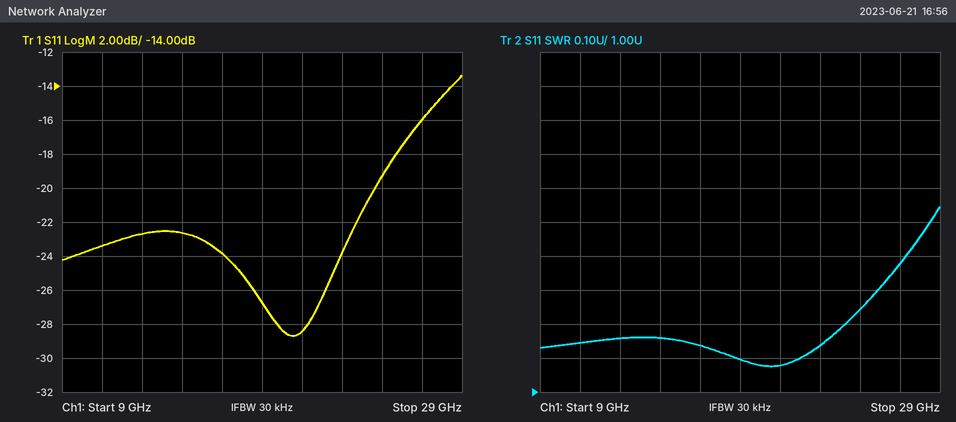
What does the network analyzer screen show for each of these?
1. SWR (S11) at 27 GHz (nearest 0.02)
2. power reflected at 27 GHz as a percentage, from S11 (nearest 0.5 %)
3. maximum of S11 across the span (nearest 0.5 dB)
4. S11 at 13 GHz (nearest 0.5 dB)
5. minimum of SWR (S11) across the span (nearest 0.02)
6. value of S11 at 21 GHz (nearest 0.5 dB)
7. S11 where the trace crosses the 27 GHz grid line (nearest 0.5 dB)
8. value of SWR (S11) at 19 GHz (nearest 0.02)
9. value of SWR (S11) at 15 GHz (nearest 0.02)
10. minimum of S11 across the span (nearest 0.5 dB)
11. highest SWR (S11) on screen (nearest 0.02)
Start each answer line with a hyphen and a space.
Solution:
- 1.38
- 2.5 %
- -13.5 dB
- -22.5 dB
- 1.08
- -28.5 dB
- -16.0 dB
- 1.10
- 1.16
- -28.5 dB
- 1.54
